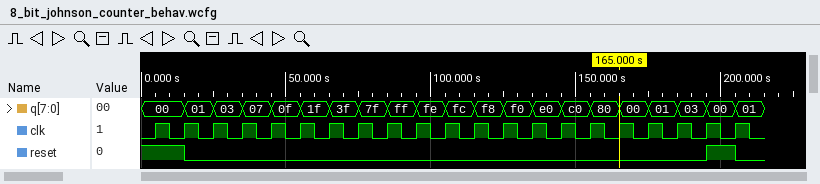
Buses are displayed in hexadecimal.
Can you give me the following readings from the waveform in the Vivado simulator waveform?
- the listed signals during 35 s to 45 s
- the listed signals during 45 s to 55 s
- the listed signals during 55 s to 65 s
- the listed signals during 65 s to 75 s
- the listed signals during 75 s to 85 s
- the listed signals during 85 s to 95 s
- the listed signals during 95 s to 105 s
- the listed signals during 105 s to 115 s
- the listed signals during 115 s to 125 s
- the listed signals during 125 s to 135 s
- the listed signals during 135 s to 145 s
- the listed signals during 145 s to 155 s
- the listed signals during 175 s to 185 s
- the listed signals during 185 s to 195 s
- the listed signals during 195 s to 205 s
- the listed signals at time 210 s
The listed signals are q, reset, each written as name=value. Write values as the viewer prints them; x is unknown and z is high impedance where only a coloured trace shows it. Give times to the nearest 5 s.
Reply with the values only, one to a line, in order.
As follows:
q=07, reset=0
q=0f, reset=0
q=1f, reset=0
q=3f, reset=0
q=7f, reset=0
q=ff, reset=0
q=fe, reset=0
q=fc, reset=0
q=f8, reset=0
q=f0, reset=0
q=e0, reset=0
q=c0, reset=0
q=01, reset=0
q=03, reset=0
q=00, reset=1
q=01, reset=0
